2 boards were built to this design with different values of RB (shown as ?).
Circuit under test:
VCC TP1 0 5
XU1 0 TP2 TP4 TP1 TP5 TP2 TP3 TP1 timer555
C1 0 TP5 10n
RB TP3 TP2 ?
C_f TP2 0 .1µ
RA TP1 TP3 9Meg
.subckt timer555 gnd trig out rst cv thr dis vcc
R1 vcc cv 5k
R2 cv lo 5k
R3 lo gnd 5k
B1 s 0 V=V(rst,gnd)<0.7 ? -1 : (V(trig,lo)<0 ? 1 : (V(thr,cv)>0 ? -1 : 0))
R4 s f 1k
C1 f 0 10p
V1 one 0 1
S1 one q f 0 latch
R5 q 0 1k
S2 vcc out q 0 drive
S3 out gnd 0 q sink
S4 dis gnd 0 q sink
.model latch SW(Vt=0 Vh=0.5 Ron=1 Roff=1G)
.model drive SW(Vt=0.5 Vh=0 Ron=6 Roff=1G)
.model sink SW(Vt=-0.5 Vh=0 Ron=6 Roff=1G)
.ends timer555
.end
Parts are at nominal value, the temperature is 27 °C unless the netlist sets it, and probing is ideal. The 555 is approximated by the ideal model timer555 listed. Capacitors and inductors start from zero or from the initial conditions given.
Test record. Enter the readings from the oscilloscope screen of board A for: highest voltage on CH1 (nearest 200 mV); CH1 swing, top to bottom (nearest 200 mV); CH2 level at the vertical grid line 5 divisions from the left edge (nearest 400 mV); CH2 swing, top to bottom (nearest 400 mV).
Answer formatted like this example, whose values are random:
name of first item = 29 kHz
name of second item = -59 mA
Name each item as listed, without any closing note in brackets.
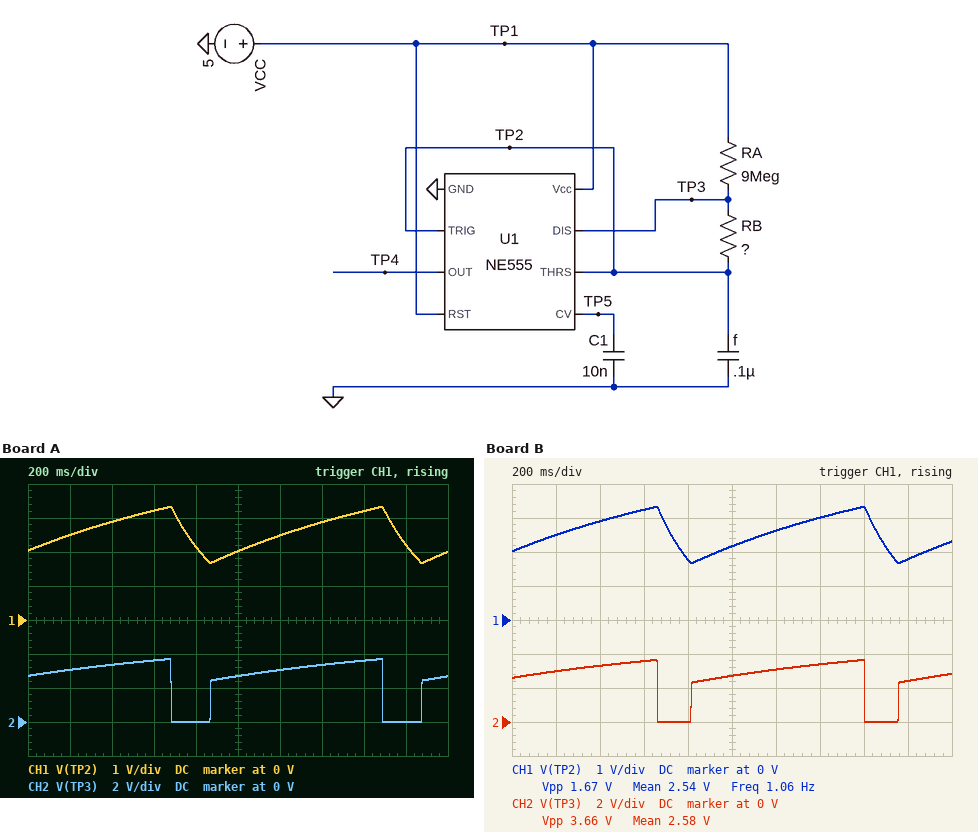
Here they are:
highest voltage on CH1 = 3.4 V
CH1 swing, top to bottom = 1.6 V
CH2 level at the vertical grid line 5 divisions from the left edge = 2.8 V
CH2 swing, top to bottom = 3.6 V
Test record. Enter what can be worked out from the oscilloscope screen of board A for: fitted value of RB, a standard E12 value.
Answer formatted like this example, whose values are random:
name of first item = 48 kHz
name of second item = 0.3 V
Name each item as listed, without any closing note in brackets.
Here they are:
fitted value of RB, a standard E12 value = 2.7 MΩ
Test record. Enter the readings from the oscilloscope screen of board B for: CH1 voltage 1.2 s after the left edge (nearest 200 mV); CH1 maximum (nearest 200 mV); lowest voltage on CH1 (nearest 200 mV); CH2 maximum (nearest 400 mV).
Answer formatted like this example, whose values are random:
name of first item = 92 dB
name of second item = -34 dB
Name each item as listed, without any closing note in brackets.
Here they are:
CH1 voltage 1.2 s after the left edge = 2.6 V
CH1 maximum = 3.4 V
lowest voltage on CH1 = 1.6 V
CH2 maximum = 3.6 V
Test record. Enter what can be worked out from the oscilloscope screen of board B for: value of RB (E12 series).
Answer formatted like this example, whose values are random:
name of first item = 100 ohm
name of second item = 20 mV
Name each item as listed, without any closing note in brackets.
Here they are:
value of RB = 2.2 MΩ
